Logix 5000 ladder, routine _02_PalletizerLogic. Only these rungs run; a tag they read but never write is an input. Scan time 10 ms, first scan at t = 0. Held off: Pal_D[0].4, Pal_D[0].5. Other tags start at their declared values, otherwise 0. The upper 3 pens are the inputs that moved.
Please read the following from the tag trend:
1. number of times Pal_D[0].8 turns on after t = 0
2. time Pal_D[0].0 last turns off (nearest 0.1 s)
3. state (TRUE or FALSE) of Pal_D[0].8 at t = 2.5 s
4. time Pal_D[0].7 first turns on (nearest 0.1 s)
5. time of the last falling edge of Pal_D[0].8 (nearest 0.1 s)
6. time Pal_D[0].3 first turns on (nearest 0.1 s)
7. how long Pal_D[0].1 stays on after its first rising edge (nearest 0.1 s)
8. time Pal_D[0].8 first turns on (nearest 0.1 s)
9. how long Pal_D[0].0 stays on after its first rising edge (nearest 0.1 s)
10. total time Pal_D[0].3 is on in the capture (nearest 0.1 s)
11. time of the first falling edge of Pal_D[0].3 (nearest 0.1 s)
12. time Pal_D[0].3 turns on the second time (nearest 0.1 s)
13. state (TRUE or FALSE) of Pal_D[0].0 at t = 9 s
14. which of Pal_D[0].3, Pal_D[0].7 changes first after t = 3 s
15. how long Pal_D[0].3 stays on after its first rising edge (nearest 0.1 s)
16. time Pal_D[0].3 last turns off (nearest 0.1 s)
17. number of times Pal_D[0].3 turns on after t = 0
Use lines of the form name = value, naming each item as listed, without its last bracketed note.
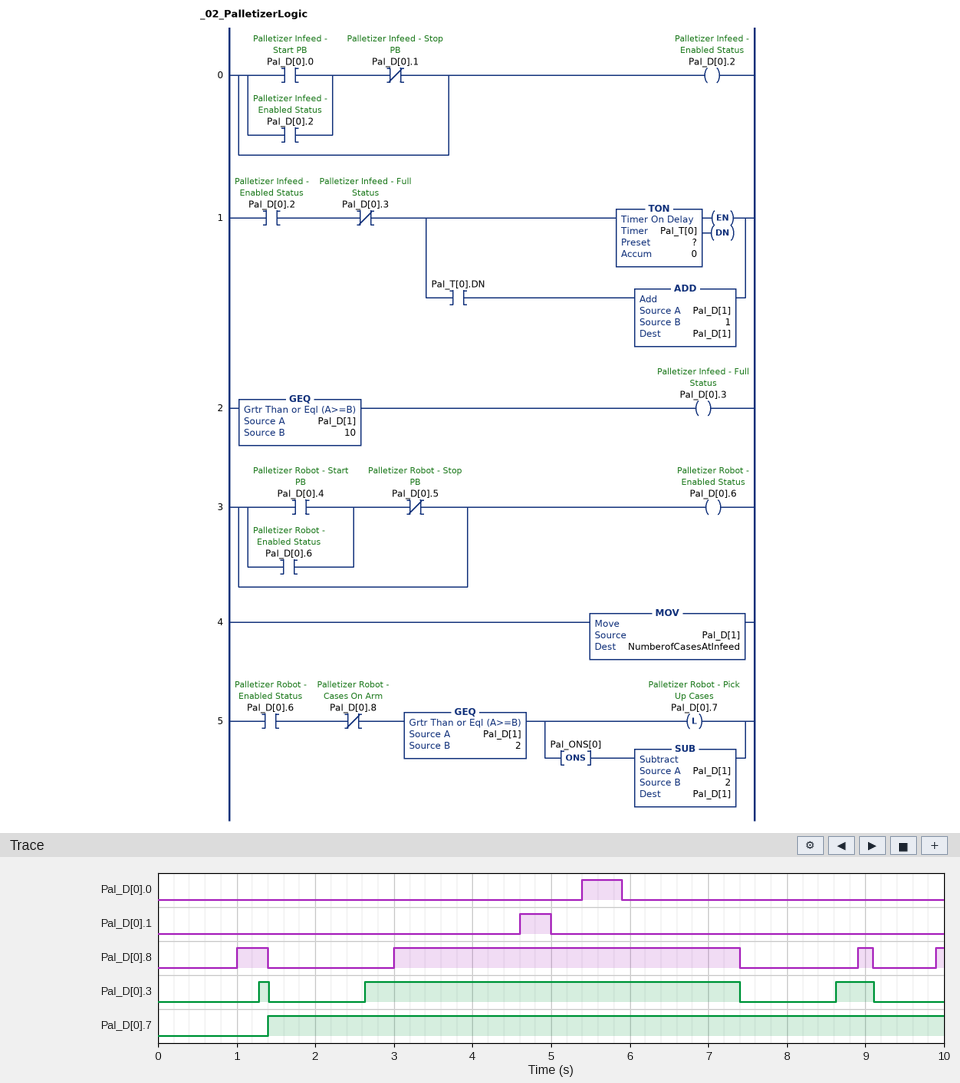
number of times Pal_D[0].8 turns on after t = 0 = 4
time Pal_D[0].0 last turns off = 5.9 s
state (TRUE or FALSE) of Pal_D[0].8 at t = 2.5 s = FALSE
time Pal_D[0].7 first turns on = 1.4 s
time of the last falling edge of Pal_D[0].8 = 9.1 s
time Pal_D[0].3 first turns on = 1.3 s
how long Pal_D[0].1 stays on after its first rising edge = 0.4 s
time Pal_D[0].8 first turns on = 1.0 s
how long Pal_D[0].0 stays on after its first rising edge = 0.5 s
total time Pal_D[0].3 is on in the capture = 5.4 s
time of the first falling edge of Pal_D[0].3 = 1.4 s
time Pal_D[0].3 turns on the second time = 2.6 s
state (TRUE or FALSE) of Pal_D[0].0 at t = 9 s = FALSE
which of Pal_D[0].3, Pal_D[0].7 changes first after t = 3 s = Pal_D[0].3
how long Pal_D[0].3 stays on after its first rising edge = 0.1 s
time Pal_D[0].3 last turns off = 9.1 s
number of times Pal_D[0].3 turns on after t = 0 = 3
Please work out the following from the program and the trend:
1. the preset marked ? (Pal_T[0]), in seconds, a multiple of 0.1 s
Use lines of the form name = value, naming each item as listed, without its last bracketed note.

the preset marked ? (Pal_T[0]), in seconds, a multiple of 0.1 s = 1.2 s
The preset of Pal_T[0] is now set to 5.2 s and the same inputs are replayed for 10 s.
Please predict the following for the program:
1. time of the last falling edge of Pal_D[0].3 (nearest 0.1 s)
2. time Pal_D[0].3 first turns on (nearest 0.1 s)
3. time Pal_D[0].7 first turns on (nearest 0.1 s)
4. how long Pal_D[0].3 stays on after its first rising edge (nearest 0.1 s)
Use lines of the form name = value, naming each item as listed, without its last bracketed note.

time of the last falling edge of Pal_D[0].3 = 7.4 s
time Pal_D[0].3 first turns on = 5.3 s
time Pal_D[0].7 first turns on = 7.4 s
how long Pal_D[0].3 stays on after its first rising edge = 2.1 s
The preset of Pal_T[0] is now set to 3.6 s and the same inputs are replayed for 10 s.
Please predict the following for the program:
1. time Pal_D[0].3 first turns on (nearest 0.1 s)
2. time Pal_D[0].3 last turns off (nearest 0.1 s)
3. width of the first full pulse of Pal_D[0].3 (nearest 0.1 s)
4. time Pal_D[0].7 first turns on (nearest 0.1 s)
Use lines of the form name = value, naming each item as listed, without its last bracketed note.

time Pal_D[0].3 first turns on = 3.7 s
time Pal_D[0].3 last turns off = 7.4 s
width of the first full pulse of Pal_D[0].3 = 3.7 s
time Pal_D[0].7 first turns on = 7.4 s
